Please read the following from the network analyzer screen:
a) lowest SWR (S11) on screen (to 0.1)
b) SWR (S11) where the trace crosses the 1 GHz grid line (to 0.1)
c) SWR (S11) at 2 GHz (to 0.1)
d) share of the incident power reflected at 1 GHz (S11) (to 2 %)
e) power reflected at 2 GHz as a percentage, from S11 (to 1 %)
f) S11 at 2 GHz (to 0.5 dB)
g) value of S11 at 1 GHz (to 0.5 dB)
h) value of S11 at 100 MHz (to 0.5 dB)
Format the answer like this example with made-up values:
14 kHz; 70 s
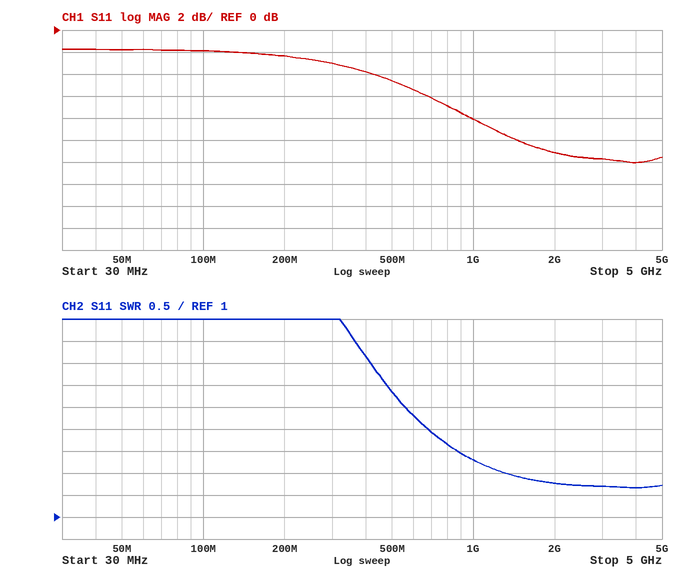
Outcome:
1.7; 2.3; 1.8; 16 %; 8 %; -11.0 dB; -8.0 dB; -2.0 dB
